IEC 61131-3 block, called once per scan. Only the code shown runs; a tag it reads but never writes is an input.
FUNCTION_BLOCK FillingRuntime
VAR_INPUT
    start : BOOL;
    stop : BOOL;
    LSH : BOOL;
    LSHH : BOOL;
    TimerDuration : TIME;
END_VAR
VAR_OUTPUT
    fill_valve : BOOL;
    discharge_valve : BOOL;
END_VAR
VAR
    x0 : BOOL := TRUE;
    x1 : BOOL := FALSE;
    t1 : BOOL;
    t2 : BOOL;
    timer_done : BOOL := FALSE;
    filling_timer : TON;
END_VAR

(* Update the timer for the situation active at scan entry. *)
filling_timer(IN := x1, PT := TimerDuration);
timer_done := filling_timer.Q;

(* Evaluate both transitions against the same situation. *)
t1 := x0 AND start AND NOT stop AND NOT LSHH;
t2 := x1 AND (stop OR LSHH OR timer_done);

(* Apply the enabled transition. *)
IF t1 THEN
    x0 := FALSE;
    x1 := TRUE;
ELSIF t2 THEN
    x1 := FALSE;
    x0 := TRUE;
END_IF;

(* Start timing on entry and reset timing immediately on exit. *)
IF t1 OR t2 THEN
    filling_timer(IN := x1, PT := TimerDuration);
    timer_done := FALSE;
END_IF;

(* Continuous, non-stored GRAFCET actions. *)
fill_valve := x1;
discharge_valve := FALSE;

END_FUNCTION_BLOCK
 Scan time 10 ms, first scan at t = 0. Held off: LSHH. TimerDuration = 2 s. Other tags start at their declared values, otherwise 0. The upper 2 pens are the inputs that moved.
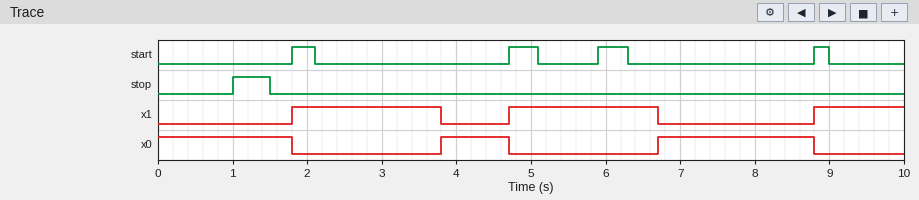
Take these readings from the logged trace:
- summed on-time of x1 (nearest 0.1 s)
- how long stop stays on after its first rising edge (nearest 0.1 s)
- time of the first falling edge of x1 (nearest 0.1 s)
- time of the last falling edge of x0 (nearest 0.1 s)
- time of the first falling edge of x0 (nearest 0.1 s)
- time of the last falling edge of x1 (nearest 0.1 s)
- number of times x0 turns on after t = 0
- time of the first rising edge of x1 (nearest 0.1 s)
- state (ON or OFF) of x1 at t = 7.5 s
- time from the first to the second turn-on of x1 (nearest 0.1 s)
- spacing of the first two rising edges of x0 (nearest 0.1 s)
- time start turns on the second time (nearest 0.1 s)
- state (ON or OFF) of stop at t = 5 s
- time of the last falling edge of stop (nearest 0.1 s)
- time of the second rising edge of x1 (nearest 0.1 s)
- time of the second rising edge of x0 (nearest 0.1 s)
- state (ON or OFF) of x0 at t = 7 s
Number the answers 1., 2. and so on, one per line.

1. 5.2 s
2. 0.5 s
3. 3.8 s
4. 8.8 s
5. 1.8 s
6. 6.7 s
7. 2
8. 1.8 s
9. OFF
10. 2.9 s
11. 2.9 s
12. 4.7 s
13. OFF
14. 1.5 s
15. 4.7 s
16. 6.7 s
17. ON
